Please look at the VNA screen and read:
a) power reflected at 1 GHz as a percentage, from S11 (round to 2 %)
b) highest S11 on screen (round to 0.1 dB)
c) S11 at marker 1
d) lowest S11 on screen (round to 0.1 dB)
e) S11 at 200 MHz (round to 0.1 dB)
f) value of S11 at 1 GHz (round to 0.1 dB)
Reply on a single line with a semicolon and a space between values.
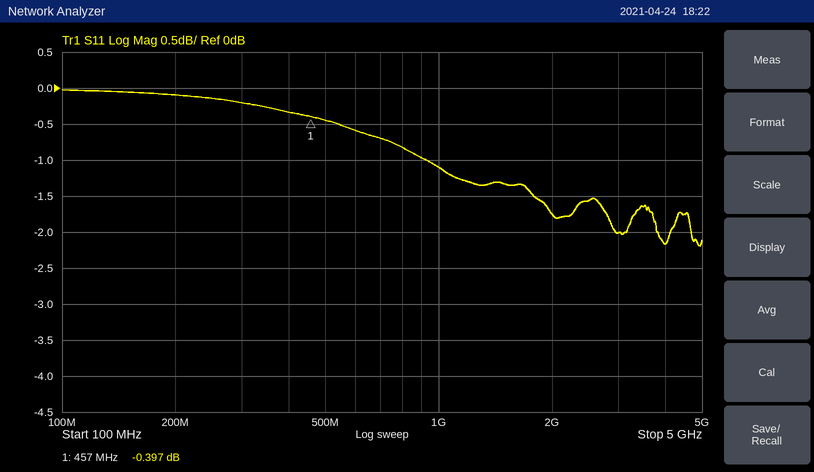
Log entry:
78 %; 0.0 dB; -0.397 dB; -2.2 dB; -0.1 dB; -1.1 dB
